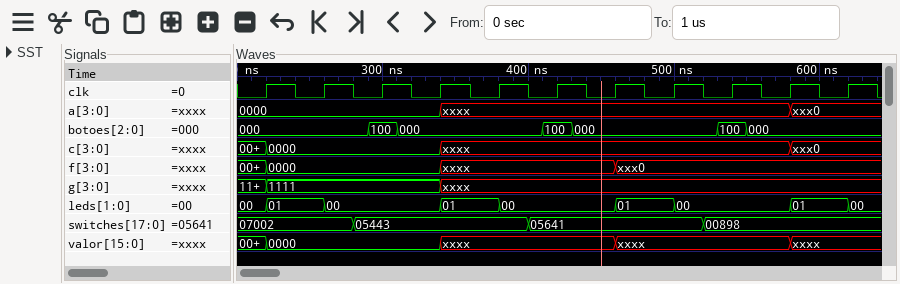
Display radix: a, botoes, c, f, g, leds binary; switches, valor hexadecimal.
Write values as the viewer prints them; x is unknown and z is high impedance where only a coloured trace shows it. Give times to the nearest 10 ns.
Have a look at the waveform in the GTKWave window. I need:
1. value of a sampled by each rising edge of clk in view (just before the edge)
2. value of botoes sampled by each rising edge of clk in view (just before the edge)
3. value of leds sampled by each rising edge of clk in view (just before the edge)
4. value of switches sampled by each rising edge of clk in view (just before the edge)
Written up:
0000, 0000, 0000, 0000, xxxx, xxxx, xxxx, xxxx, xxxx, xxxx, xxx0
000, 000, 100, 000, 000, 100, 000, 000, 100, 000, 000
00, 01, 00, 00, 01, 00, 00, 01, 00, 00, 01
07002, 07002, 05443, 05443, 05443, 05641, 05641, 05641, 00898, 00898, 00898
